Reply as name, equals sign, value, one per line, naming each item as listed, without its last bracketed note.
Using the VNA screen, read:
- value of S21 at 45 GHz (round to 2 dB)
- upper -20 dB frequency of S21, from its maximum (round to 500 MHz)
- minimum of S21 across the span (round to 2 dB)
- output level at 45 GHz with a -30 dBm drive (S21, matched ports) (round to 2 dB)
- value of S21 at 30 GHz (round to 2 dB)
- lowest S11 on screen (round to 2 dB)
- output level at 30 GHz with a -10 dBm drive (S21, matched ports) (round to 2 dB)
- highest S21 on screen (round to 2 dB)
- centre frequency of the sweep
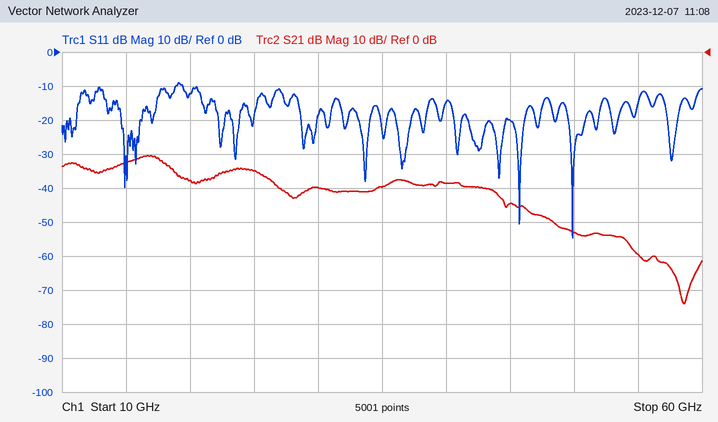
value of S21 at 45 GHz = -44 dB
upper -20 dB frequency of S21, from its maximum = 48.5 GHz
minimum of S21 across the span = -74 dB
output level at 45 GHz with a -30 dBm drive (S21, matched ports) = -74 dBm
value of S21 at 30 GHz = -40 dB
lowest S11 on screen = -54 dB
output level at 30 GHz with a -10 dBm drive (S21, matched ports) = -50 dBm
highest S21 on screen = -30 dB
centre frequency of the sweep = 35 GHz
